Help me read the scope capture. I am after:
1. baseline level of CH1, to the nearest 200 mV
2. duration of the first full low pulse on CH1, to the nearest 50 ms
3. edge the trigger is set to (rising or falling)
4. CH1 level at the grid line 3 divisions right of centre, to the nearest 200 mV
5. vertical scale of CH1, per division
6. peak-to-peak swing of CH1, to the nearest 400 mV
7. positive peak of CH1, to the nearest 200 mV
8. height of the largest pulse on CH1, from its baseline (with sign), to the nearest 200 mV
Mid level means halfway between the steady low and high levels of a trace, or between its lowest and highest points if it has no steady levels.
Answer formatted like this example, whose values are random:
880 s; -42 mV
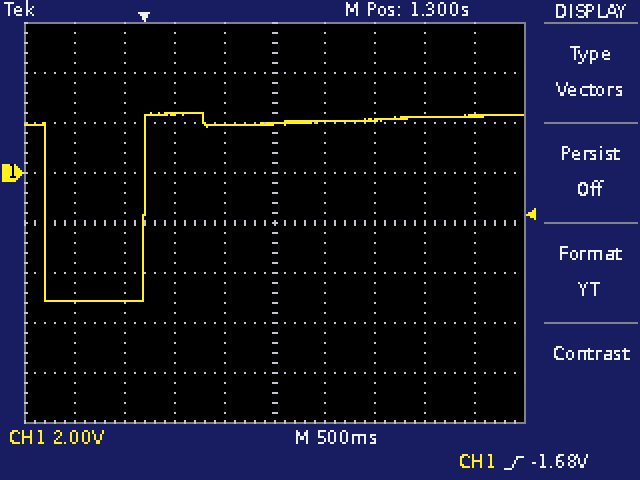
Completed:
2.0 V; 1.00 s; rising; 2.2 V; 2 V; 7.6 V; 2.4 V; -7.2 V
